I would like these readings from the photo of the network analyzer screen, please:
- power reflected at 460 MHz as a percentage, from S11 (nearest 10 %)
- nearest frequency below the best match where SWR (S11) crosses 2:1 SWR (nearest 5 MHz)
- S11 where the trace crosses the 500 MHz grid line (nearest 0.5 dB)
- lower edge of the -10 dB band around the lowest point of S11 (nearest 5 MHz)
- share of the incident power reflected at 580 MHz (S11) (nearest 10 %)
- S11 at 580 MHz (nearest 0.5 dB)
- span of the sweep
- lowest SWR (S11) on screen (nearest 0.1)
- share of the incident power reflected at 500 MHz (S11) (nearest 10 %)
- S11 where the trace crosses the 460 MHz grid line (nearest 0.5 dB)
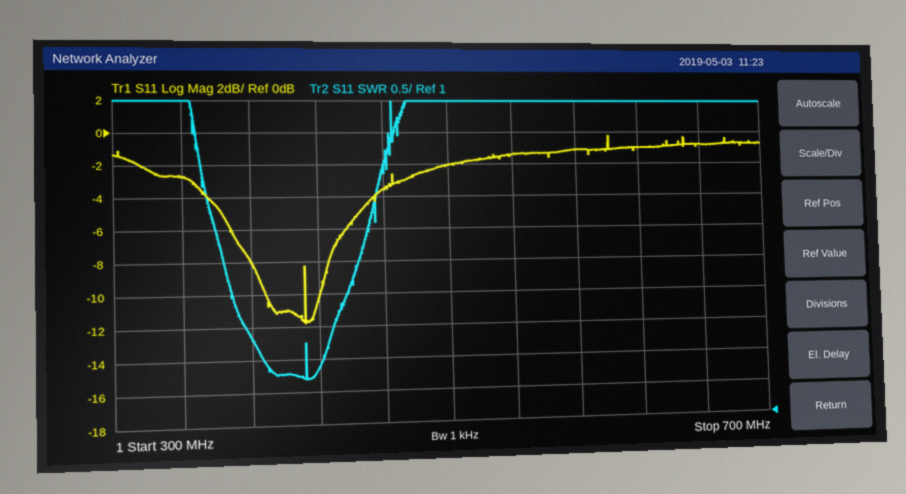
40 %
385 MHz
-2.0 dB
390 MHz
80 %
-1.0 dB
400 MHz
1.7
60 %
-3.5 dB
